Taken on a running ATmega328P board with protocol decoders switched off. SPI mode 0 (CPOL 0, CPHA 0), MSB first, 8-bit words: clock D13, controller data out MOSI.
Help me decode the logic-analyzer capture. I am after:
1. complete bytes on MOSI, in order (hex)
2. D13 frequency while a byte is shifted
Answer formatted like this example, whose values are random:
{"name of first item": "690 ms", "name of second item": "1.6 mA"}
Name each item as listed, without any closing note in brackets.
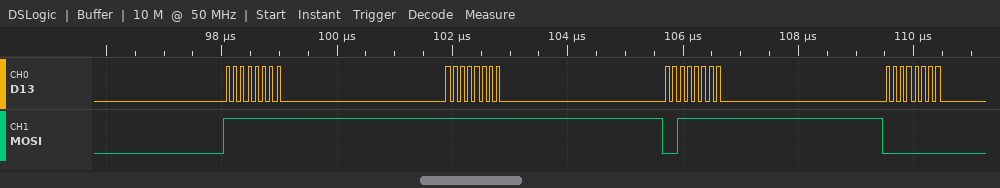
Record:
{"complete bytes on MOSI, in order": "FF FF 3F 00", "D13 frequency while a byte is shifted": "8 MHz"}
